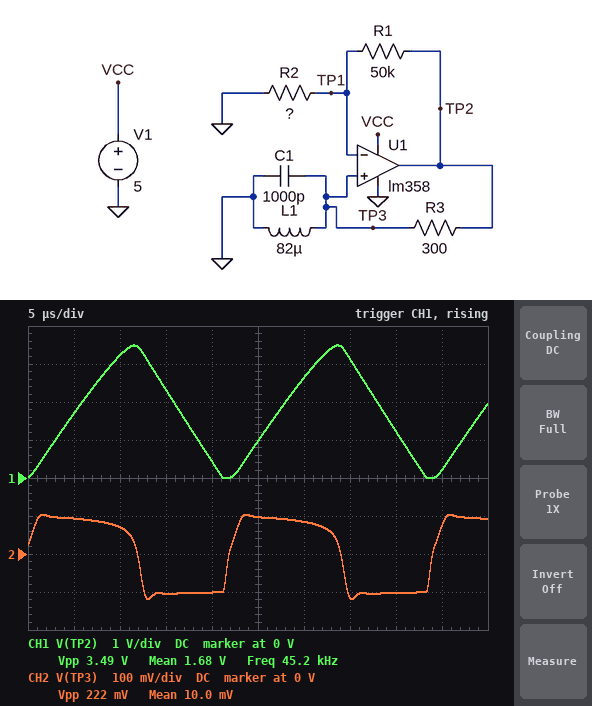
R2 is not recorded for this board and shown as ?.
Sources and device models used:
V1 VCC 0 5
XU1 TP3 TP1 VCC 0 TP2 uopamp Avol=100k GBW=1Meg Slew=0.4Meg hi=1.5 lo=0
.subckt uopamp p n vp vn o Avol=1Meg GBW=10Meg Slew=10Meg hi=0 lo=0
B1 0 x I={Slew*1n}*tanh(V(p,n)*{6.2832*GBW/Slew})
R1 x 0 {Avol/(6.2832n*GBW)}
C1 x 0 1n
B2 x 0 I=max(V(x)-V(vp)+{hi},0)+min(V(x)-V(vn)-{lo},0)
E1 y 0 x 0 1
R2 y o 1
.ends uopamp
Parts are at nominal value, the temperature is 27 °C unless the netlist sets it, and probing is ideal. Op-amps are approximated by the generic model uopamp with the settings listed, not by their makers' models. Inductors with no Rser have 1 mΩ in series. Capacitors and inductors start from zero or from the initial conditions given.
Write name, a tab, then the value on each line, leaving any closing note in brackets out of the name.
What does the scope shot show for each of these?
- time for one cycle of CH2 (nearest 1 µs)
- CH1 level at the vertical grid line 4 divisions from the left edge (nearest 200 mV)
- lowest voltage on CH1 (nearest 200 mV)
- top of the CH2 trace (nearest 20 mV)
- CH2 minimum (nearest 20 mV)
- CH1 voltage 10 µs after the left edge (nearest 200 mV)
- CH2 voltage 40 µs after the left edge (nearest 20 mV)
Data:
time for one cycle of CH2	22 µs
CH1 level at the vertical grid line 4 divisions from the left edge	400 mV
lowest voltage on CH1	0 V
top of the CH2 trace	100 mV
CH2 minimum	-120 mV
CH1 voltage 10 µs after the left edge	3.2 V
CH2 voltage 40 µs after the left edge	-100 mV
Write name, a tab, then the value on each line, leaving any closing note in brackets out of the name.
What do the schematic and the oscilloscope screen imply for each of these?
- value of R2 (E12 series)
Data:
value of R2	390 Ω
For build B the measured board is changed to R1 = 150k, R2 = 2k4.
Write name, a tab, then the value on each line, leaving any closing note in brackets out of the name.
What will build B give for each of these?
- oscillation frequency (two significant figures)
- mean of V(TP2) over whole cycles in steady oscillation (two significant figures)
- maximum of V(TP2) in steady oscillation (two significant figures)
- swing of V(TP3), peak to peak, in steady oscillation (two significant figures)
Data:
oscillation frequency	77 kHz
mean of V(TP2) over whole cycles in steady oscillation	950 mV
maximum of V(TP2) in steady oscillation	1.9 V
swing of V(TP3), peak to peak, in steady oscillation	220 mV
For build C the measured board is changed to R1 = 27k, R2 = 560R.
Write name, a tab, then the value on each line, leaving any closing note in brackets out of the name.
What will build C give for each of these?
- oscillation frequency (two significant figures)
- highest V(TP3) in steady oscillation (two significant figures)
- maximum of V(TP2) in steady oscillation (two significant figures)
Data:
oscillation frequency	92 kHz
highest V(TP3) in steady oscillation	100 mV
maximum of V(TP2) in steady oscillation	1.5 V
